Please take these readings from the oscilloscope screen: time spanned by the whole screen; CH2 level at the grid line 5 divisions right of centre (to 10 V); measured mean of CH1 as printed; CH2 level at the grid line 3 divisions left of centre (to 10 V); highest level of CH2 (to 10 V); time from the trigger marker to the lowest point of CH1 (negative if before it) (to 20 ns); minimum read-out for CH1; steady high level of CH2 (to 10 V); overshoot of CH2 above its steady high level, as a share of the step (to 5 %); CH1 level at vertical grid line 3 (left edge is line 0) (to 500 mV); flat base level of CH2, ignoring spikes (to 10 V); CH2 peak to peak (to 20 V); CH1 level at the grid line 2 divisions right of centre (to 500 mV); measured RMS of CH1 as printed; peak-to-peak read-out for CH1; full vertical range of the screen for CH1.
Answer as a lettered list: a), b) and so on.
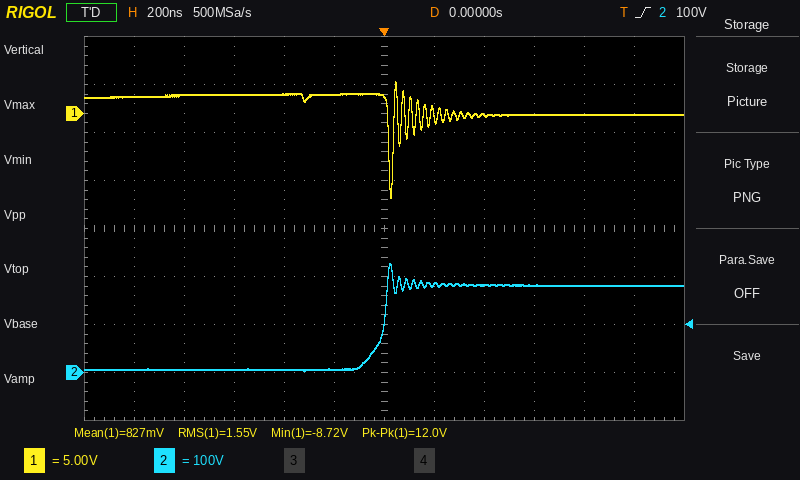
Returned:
a) 2.4 µs
b) 180 V
c) 827 mV
d) 10 V
e) 230 V
f) +20 ns
g) -8.72 V
h) 180 V
i) 25 %
j) 2.0 V
k) 10 V
l) 220 V
m) 0.0 V
n) 1.55 V
o) 12.0 V
p) 40 V
